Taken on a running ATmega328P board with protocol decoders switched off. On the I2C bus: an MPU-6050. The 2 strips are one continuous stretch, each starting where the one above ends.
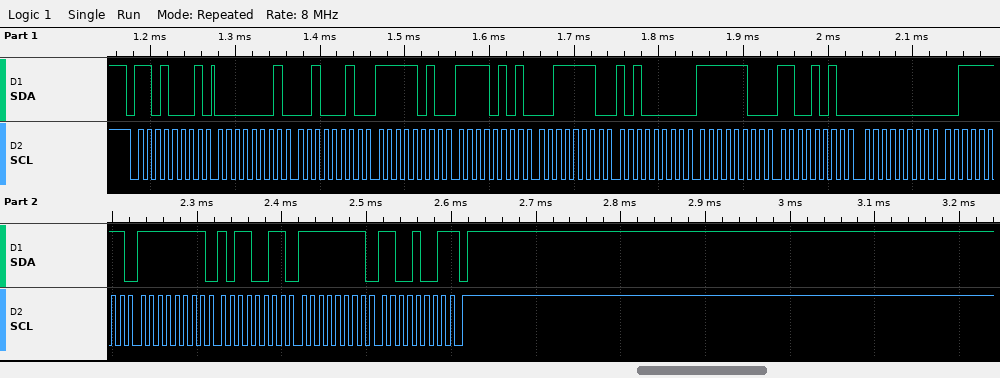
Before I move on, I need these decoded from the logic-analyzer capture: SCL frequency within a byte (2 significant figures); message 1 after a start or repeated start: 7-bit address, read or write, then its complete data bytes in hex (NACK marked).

100 kHz
0x68 read: 01 22 FA F5 3E A0 FC CA 00 3F FF B3 FF C9 NACK
